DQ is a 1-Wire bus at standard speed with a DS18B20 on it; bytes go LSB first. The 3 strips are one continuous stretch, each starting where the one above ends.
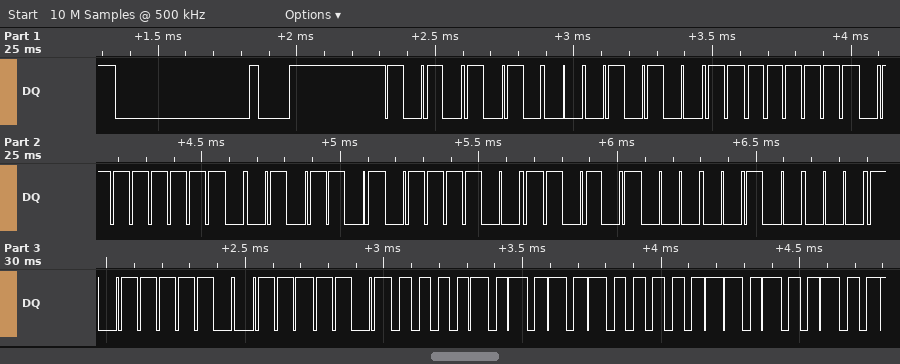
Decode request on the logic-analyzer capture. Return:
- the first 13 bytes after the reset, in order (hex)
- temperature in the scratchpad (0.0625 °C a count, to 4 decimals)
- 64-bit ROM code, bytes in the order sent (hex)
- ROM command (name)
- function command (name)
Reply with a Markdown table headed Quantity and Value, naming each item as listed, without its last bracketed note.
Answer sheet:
| Quantity | Value |
|---|---|
| the first 13 bytes after the reset, in order | 55 28 FF FE B4 9E 15 04 7D BE 50 05 4B |
| temperature in the scratchpad | 85.0000 °C |
| 64-bit ROM code, bytes in the order sent | 28 FF FE B4 9E 15 04 7D |
| ROM command | Match ROM |
| function command | Read Scratchpad |
